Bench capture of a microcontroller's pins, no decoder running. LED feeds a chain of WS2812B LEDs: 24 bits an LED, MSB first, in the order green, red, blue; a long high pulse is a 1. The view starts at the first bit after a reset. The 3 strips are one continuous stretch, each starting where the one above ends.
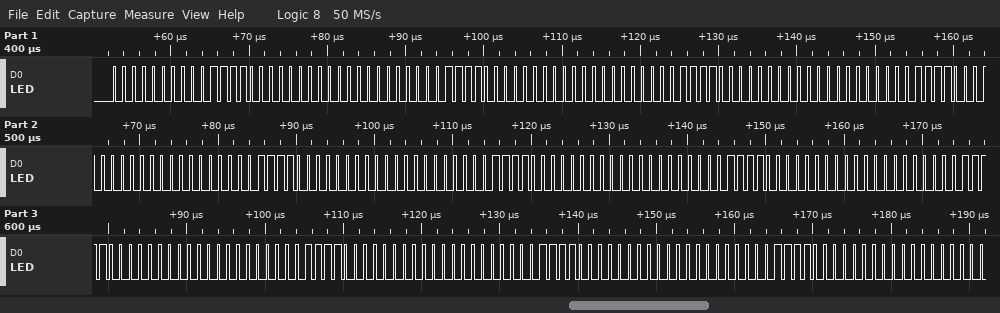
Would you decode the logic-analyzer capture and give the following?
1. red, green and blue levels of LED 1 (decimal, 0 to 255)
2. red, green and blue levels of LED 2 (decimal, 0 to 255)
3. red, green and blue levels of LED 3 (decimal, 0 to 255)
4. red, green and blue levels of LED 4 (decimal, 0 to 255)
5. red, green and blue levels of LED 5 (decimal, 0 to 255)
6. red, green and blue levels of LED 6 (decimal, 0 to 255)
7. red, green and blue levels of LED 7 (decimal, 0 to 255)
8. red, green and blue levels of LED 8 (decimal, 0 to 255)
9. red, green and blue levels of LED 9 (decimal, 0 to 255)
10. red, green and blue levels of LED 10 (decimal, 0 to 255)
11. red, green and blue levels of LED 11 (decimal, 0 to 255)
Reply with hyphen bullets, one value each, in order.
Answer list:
- 60, 0, 0
- 60, 0, 0
- 60, 0, 0
- 60, 0, 0
- 60, 0, 0
- 60, 0, 0
- 60, 0, 0
- 60, 0, 0
- 60, 0, 0
- 60, 0, 0
- 60, 0, 0
